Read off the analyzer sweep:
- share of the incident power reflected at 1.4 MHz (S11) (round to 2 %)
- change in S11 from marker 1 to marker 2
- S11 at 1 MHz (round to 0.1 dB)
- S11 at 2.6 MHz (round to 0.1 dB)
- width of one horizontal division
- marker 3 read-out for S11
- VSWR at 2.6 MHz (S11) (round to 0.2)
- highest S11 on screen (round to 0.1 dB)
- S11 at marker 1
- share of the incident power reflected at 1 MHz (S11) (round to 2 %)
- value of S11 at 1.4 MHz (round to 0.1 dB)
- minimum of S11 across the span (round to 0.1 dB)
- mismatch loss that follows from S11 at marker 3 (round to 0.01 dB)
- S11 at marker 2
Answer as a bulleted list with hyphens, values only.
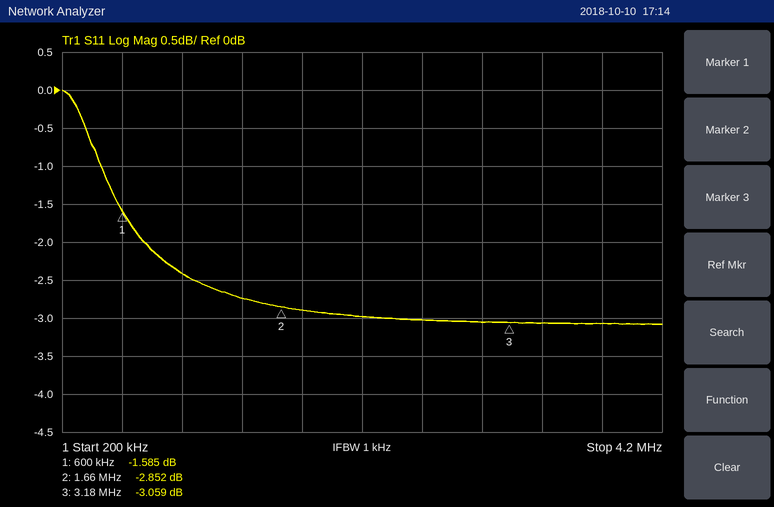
- 54 %
- -1.267 dB
- -2.4 dB
- -3.0 dB
- 400 kHz
- -3.059 dB
- 5.8
- 0.0 dB
- -1.585 dB
- 58 %
- -2.7 dB
- -3.1 dB
- 2.96 dB
- -2.852 dB
